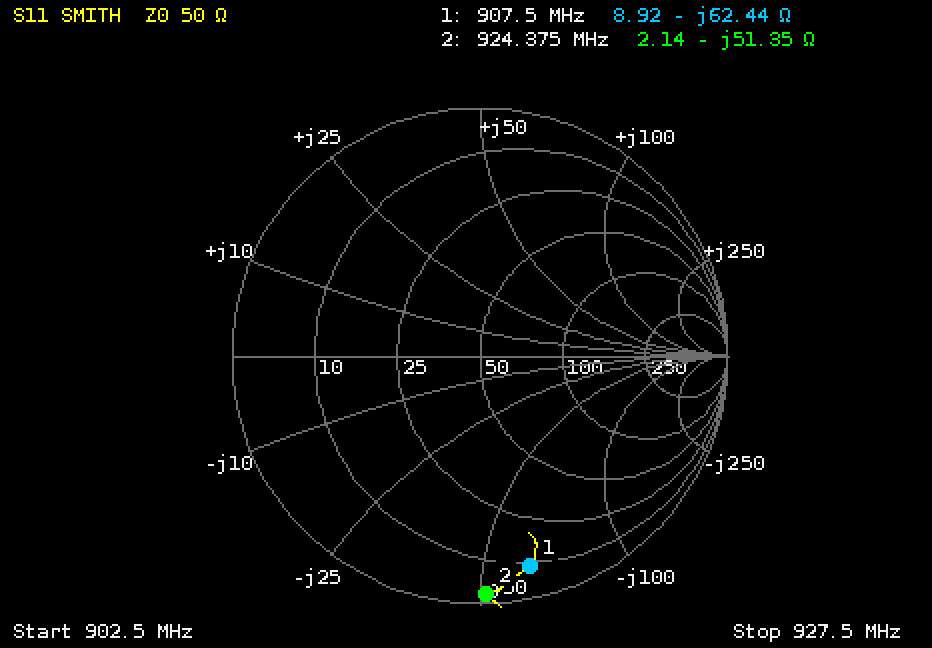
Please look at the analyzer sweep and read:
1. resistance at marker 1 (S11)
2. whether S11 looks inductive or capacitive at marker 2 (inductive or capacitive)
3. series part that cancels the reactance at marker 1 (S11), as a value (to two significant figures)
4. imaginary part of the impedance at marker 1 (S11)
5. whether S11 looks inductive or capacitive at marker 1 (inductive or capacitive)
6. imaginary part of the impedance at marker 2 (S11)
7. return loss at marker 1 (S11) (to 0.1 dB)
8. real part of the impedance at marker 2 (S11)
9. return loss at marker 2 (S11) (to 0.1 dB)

8.92 Ω
capacitive
11 nH
-62.44 Ω
capacitive
-51.35 Ω
1.2 dB
2.14 Ω
0.4 dB
